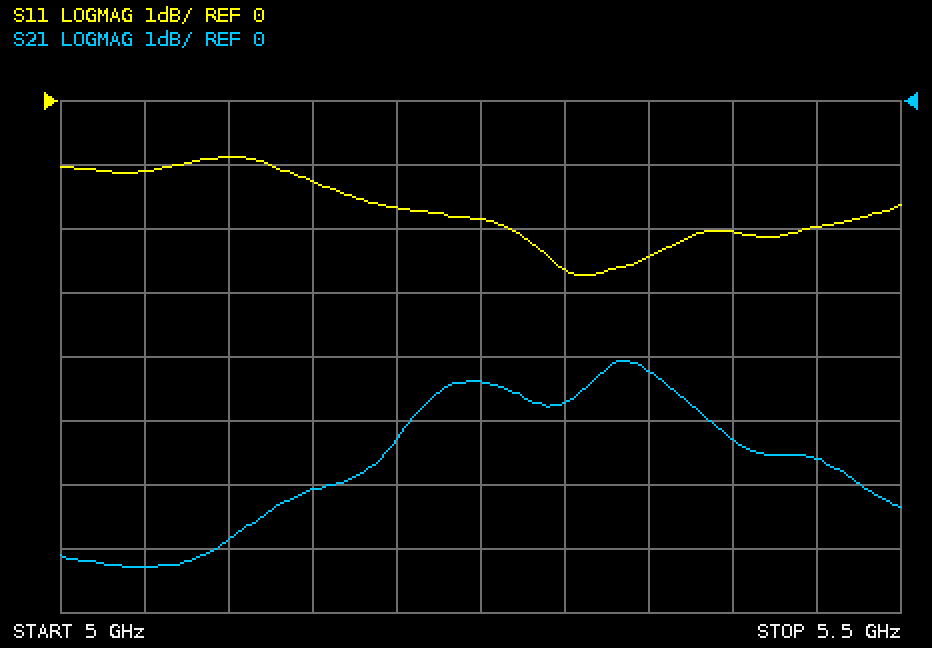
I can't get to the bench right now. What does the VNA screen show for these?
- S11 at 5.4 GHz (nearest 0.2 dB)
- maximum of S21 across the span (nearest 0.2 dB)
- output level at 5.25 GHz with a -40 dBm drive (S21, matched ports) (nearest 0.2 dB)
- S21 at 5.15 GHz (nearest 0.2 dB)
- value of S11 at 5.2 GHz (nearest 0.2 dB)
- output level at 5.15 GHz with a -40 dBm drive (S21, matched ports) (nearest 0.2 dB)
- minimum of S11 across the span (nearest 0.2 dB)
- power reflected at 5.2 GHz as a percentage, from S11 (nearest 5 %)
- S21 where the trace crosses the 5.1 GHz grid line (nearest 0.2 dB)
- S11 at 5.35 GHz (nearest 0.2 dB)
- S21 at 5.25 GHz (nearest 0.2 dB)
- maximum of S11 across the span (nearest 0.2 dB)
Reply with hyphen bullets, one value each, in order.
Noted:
- -2.0 dB
- -4.0 dB
- -44.4 dBm
- -6.0 dB
- -1.6 dB
- -46.0 dBm
- -2.8 dB
- 70 %
- -6.8 dB
- -2.4 dB
- -4.4 dB
- -0.8 dB
